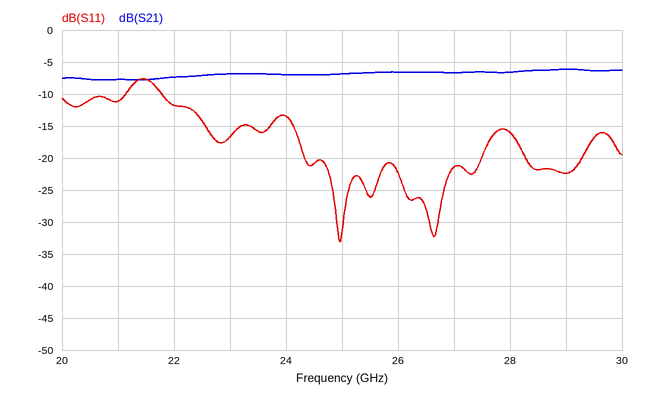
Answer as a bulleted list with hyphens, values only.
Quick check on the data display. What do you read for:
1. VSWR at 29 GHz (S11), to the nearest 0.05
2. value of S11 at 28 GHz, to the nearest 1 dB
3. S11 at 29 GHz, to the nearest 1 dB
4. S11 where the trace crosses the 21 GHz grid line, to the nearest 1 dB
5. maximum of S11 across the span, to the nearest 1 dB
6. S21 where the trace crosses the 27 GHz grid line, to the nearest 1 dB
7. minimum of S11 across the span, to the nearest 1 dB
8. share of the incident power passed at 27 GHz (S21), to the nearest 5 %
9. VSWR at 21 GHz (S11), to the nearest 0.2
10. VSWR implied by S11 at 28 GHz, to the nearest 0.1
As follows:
- 1.15
- -16 dB
- -22 dB
- -11 dB
- -8 dB
- -7 dB
- -33 dB
- 20 %
- 1.8
- 1.4
